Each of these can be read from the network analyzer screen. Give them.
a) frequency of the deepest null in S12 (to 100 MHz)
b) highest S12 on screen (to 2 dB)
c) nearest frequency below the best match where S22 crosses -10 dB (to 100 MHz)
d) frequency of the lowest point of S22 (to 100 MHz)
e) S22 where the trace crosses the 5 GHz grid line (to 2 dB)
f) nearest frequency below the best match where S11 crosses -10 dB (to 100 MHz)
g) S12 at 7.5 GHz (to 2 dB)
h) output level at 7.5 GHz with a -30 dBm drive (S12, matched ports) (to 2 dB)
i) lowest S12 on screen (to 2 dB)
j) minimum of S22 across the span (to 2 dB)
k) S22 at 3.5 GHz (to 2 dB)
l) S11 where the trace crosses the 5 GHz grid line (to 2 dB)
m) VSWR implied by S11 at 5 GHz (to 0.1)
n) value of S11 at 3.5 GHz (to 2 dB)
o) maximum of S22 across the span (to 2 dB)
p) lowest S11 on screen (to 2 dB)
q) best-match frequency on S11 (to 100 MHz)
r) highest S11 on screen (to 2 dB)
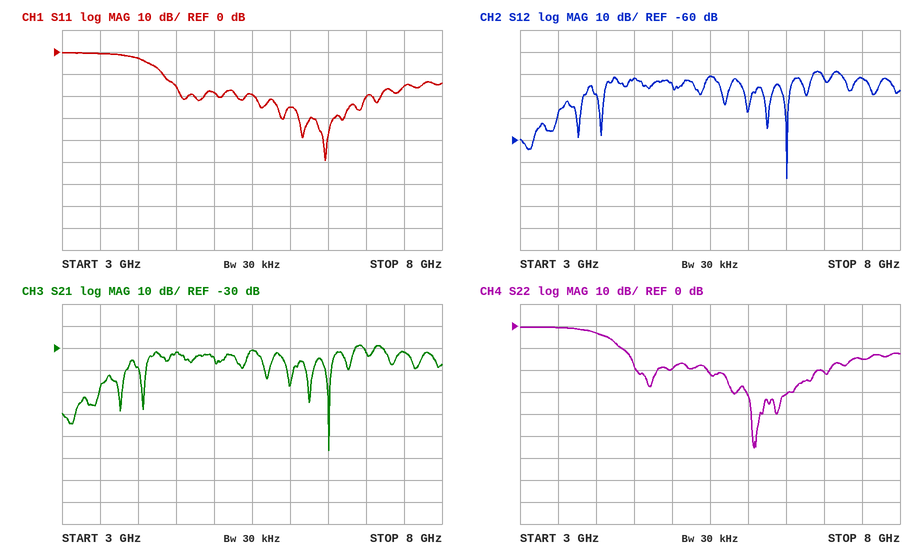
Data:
6.5 GHz
-28 dB
4.3 GHz
6.1 GHz
-20 dB
4.3 GHz
-32 dB
-62 dBm
-78 dB
-56 dB
0 dB
-18 dB
1.3
0 dB
0 dB
-50 dB
6.5 GHz
0 dB
